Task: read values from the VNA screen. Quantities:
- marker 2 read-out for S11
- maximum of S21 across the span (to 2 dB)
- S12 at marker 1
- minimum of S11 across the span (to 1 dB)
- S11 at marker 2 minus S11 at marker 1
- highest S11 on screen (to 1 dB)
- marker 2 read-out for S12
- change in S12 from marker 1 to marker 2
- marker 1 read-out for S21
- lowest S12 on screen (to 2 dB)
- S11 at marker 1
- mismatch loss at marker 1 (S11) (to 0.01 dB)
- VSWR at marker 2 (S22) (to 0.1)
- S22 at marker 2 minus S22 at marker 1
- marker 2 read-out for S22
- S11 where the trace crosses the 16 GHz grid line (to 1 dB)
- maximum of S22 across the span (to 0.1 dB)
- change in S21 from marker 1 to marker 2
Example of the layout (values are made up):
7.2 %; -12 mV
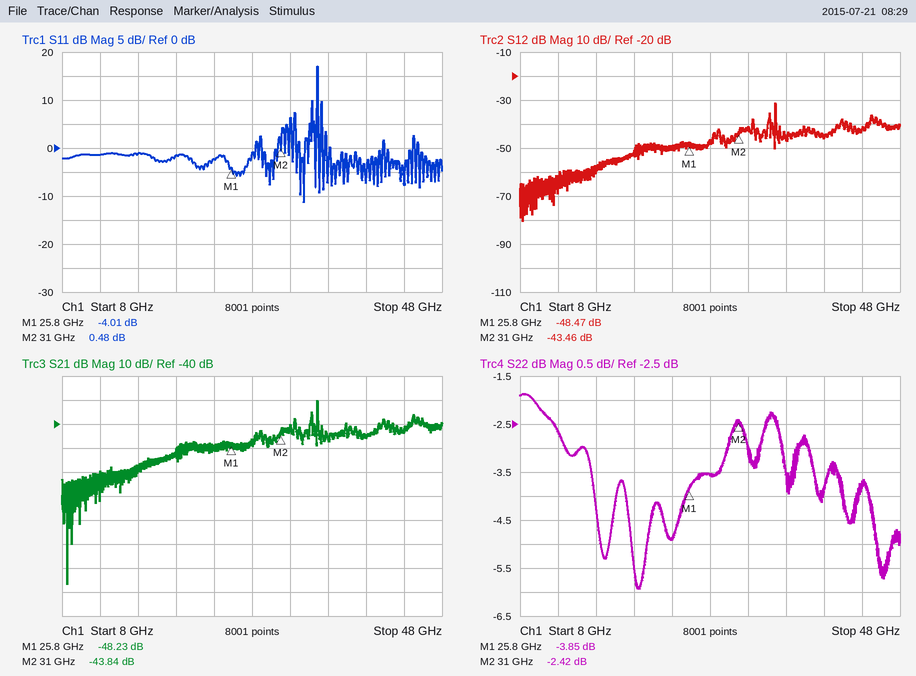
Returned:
0.48 dB; -30 dB; -48.47 dB; -11 dB; 4.49 dB; 17 dB; -43.46 dB; 5.01 dB; -48.23 dB; -80 dB; -4.01 dB; 2.20 dB; 7.2; 1.43 dB; -2.42 dB; -1 dB; -1.9 dB; 4.39 dB
